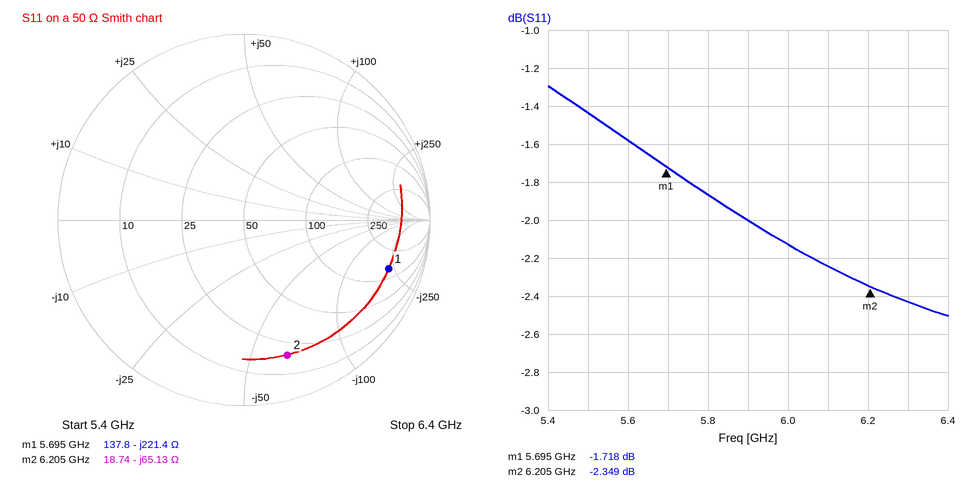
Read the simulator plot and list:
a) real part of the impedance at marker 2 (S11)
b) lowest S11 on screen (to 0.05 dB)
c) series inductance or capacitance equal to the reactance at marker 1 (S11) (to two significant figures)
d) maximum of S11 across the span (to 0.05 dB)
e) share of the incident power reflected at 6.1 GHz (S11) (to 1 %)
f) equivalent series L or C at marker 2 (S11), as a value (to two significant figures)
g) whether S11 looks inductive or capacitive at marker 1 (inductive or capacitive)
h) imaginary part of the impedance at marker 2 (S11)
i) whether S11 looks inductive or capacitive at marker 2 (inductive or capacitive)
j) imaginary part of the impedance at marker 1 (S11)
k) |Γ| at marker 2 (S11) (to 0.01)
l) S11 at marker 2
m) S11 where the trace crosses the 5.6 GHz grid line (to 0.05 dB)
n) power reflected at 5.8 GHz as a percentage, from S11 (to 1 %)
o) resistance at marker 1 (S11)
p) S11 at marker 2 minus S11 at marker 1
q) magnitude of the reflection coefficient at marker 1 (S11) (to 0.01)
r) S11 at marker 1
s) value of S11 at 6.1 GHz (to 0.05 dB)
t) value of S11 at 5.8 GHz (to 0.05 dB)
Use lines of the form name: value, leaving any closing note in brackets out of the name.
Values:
real part of the impedance at marker 2: 18.74 Ω
lowest S11 on screen: -2.50 dB
series inductance or capacitance equal to the reactance at marker 1 (S11): 130 fF
maximum of S11 across the span: -1.30 dB
share of the incident power reflected at 6.1 GHz (S11): 60 %
equivalent series L or C at marker 2 (S11), as a value: 390 fF
whether S11 looks inductive or capacitive at marker 1: capacitive
imaginary part of the impedance at marker 2: -65.13 Ω
whether S11 looks inductive or capacitive at marker 2: capacitive
imaginary part of the impedance at marker 1: -221.4 Ω
|Γ| at marker 2 (S11): 0.76
S11 at marker 2: -2.349 dB
S11 where the trace crosses the 5.6 GHz grid line: -1.60 dB
power reflected at 5.8 GHz as a percentage, from S11: 65 %
resistance at marker 1: 137.8 Ω
S11 at marker 2 minus S11 at marker 1: -0.631 dB
magnitude of the reflection coefficient at marker 1 (S11): 0.82
S11 at marker 1: -1.718 dB
value of S11 at 6.1 GHz: -2.25 dB
value of S11 at 5.8 GHz: -1.85 dB
